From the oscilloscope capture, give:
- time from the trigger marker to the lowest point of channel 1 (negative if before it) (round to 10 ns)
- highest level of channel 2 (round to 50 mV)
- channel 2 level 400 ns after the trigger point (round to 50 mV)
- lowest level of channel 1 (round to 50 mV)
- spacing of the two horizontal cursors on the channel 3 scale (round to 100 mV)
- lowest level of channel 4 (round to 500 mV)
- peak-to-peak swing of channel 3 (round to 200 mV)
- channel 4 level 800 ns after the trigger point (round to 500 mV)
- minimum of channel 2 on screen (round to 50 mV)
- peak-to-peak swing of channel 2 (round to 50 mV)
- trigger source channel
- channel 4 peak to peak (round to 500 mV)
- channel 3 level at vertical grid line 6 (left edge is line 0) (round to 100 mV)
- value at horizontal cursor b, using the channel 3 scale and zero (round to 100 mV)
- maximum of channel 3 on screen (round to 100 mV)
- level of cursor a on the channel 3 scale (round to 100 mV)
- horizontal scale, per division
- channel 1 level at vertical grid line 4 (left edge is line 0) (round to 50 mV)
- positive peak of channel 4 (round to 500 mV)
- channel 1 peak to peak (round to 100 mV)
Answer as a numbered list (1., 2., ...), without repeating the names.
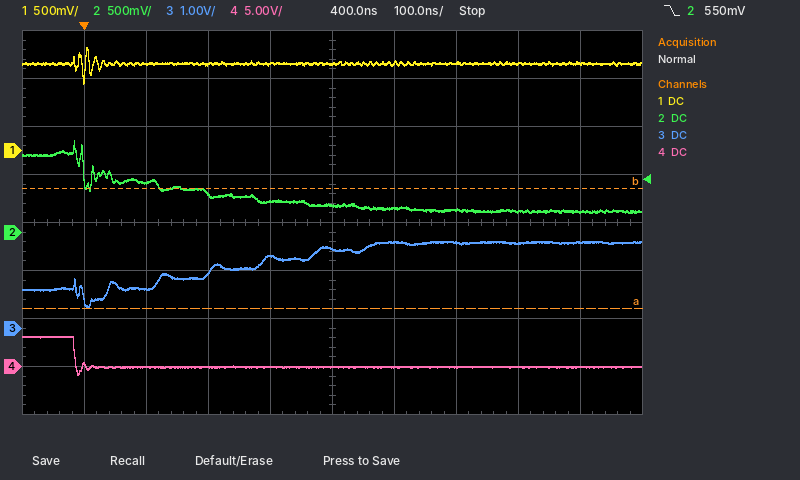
1. 0 ns
2. 950 mV
3. 300 mV
4. 700 mV
5. 2.5 V
6. -1.0 V
7. 1.4 V
8. 0.0 V
9. 200 mV
10. 750 mV
11. channel 2
12. 4.0 V
13. 1.8 V
14. 2.9 V
15. 1.8 V
16. 400 mV
17. 100 ns
18. 900 mV
19. 3.0 V
20. 400 mV
